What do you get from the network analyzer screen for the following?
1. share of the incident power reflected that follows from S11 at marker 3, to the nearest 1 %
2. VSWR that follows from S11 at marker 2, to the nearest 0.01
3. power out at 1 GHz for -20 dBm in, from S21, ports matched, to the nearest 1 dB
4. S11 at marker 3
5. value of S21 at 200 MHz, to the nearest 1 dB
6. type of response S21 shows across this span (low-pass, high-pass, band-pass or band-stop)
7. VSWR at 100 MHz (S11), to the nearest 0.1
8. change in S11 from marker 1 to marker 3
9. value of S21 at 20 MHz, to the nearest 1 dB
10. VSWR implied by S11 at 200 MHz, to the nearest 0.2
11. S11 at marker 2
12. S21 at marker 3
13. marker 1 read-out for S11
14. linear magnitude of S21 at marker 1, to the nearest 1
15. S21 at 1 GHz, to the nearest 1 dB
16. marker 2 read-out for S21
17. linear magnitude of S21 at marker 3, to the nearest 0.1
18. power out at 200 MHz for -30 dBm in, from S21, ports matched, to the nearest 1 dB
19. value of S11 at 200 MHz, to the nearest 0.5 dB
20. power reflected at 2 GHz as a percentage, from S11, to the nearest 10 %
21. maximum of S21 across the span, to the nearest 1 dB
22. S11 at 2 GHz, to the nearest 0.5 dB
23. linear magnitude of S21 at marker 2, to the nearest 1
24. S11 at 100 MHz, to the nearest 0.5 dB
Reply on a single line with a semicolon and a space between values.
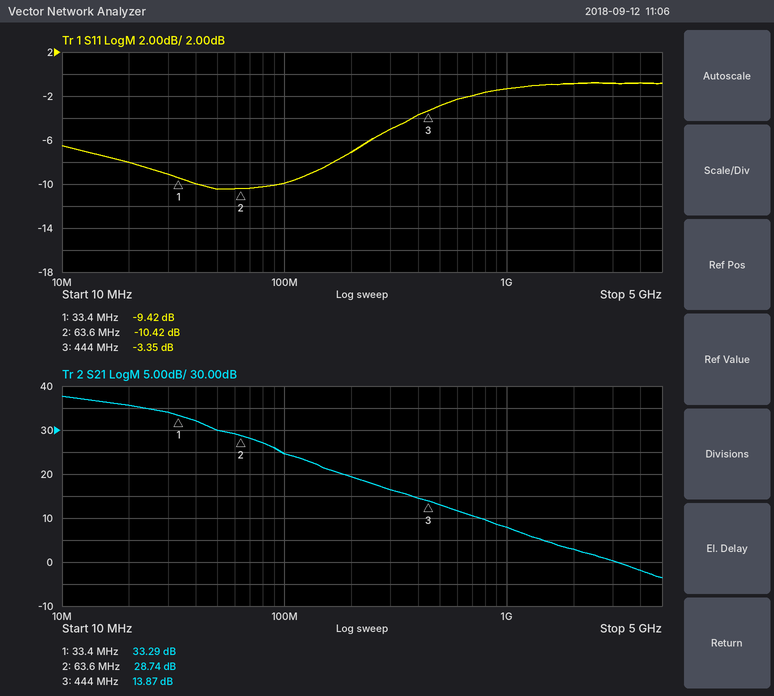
46 %; 1.86; -12 dBm; -3.35 dB; 19 dB; low-pass; 1.9; 6.07 dB; 36 dB; 2.6; -10.42 dB; 13.87 dB; -9.42 dB; 46; 8 dB; 28.74 dB; 4.9; -11 dBm; -7.0 dB; 80 %; 38 dB; -1.0 dB; 27; -10.0 dB
